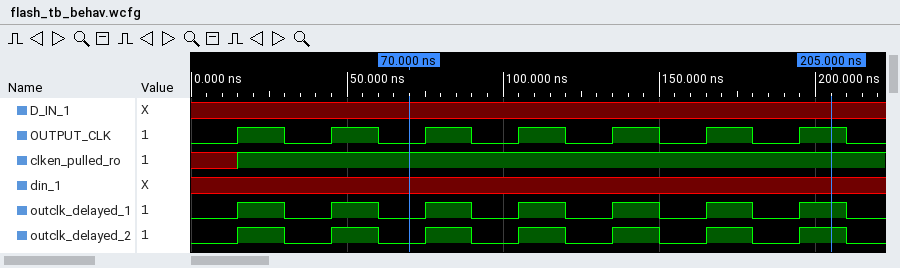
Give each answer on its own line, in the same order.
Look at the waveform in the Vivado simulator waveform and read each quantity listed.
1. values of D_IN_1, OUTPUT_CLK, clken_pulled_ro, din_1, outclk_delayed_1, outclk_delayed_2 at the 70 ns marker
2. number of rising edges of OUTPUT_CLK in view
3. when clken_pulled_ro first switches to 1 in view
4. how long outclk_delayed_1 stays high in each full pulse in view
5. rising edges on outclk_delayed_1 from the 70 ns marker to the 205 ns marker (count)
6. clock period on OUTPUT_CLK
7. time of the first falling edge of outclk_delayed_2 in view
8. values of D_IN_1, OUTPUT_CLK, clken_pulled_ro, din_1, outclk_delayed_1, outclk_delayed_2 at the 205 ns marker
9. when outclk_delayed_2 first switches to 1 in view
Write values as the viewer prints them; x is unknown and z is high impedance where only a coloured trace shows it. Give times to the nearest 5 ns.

D_IN_1=x, OUTPUT_CLK=0, clken_pulled_ro=1, din_1=x, outclk_delayed_1=0, outclk_delayed_2=0
7
15 ns
15 ns, 15 ns, 15 ns, 15 ns, 15 ns, 15 ns, 15 ns
5
30 ns
30 ns
D_IN_1=x, OUTPUT_CLK=1, clken_pulled_ro=1, din_1=x, outclk_delayed_1=1, outclk_delayed_2=1
15 ns
